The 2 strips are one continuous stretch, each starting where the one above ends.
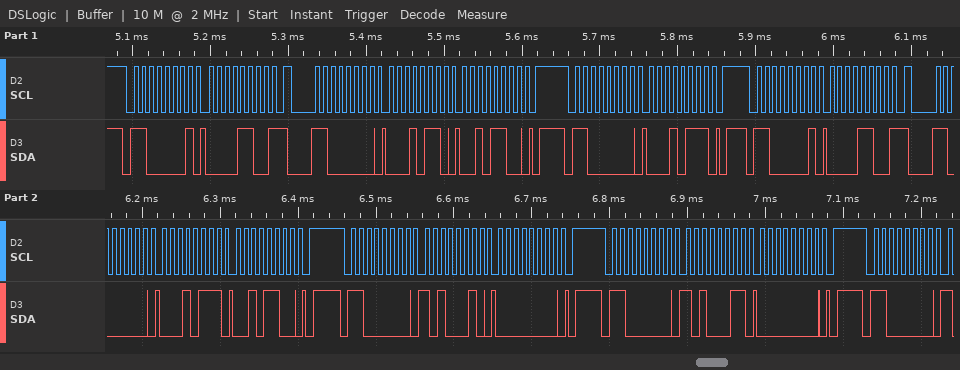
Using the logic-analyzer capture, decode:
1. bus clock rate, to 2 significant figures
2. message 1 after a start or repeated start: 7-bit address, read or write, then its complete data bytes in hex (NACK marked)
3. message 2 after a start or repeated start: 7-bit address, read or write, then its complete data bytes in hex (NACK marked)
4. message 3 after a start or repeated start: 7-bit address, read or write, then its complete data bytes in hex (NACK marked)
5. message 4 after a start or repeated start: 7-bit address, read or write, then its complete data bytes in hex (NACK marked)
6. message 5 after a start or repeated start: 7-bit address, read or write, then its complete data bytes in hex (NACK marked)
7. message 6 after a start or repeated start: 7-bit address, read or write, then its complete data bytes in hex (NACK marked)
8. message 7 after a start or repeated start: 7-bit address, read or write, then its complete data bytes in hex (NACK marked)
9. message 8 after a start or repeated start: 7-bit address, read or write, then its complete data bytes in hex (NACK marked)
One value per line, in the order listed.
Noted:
100 kHz
0x60 read: 0C NACK
0x60 write: 16 2C
0x60 write: 17
0x60 read: 0C NACK
0x60 write: 17 2C
0x60 write: A2 00
0x60 write: A3 00
0x60 write
